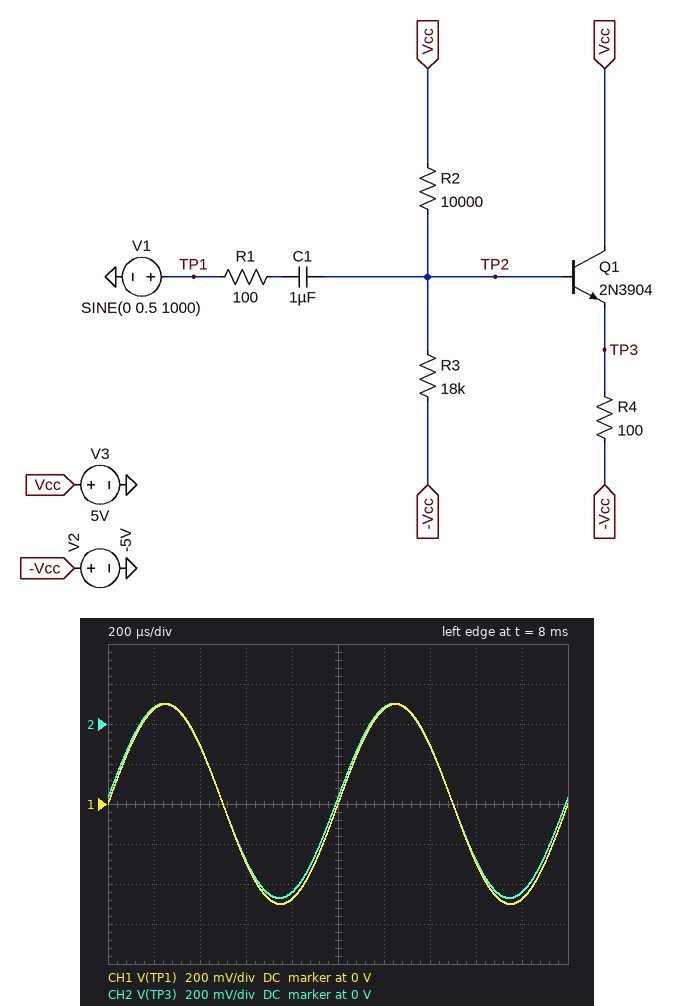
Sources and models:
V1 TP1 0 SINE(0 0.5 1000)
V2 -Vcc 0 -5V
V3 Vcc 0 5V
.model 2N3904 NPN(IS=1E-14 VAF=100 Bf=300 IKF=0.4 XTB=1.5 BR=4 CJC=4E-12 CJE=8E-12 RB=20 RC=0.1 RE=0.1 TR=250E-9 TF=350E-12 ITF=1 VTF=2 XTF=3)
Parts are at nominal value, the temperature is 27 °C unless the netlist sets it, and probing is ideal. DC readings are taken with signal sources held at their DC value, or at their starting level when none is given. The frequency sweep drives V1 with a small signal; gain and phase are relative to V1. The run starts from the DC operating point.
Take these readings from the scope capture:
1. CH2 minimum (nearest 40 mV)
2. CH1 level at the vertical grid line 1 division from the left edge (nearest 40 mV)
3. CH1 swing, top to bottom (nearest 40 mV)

-880 mV
480 mV
1.00 V
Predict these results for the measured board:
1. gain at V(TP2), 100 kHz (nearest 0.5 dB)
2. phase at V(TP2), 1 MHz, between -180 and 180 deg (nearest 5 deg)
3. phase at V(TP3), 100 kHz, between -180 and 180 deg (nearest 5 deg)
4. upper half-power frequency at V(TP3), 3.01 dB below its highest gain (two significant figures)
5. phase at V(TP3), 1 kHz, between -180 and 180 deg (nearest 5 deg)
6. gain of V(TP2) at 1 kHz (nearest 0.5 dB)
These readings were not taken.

0 dB
0 deg
0 deg
200 MHz
0 deg
0 dB
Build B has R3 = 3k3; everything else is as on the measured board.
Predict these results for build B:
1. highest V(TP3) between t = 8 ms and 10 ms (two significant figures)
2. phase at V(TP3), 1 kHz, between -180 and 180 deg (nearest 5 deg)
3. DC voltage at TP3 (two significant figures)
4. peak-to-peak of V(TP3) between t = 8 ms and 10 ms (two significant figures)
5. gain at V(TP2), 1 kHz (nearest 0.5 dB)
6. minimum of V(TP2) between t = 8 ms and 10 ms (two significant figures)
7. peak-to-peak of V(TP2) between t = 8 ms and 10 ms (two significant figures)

-2.9 V
5 deg
-3.4 V
940 mV
-0.5 dB
-3.1 V
960 mV
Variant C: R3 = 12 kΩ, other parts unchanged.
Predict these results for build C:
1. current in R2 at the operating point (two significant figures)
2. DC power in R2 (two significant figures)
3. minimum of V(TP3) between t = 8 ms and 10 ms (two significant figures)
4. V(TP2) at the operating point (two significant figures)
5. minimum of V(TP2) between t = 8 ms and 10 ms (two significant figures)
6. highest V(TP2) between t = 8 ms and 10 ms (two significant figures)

530 µA
2.8 mW
-1.5 V
-290 mV
-780 mV
200 mV
